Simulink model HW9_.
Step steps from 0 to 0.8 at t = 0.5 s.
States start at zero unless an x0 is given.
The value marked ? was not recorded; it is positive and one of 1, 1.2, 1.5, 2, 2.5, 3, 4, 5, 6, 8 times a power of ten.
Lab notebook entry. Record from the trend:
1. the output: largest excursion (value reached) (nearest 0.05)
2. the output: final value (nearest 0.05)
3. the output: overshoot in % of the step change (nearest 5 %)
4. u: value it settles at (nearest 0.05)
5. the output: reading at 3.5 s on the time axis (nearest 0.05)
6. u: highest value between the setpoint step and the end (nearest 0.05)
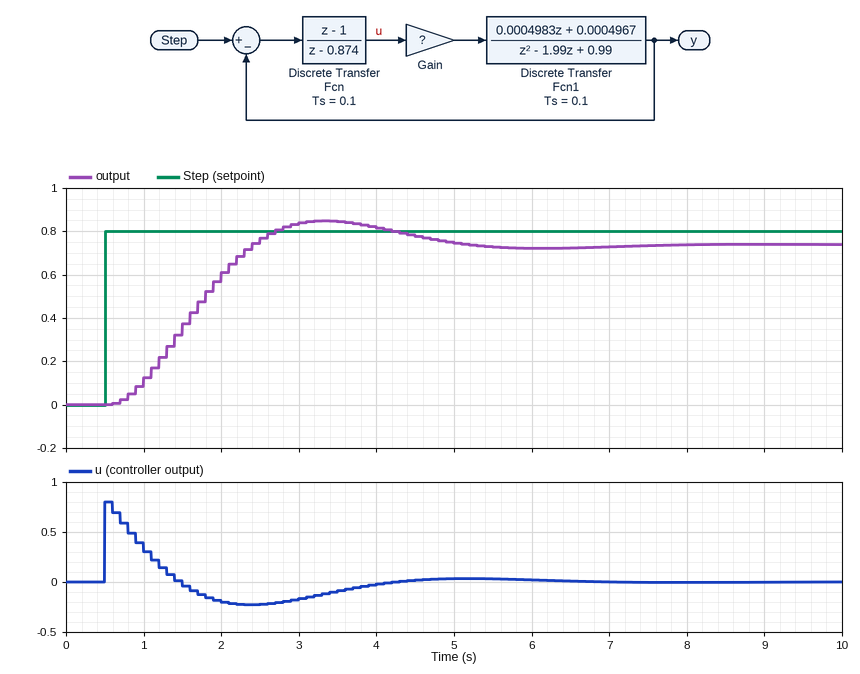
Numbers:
0.85
0.75
15 %
0.00
0.85
0.80
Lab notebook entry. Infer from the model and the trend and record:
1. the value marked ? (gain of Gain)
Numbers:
15
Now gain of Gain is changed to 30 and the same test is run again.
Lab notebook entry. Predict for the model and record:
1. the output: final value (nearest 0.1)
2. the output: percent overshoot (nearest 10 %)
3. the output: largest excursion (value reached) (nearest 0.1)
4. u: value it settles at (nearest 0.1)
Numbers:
0.8
30 %
1.0
0.0
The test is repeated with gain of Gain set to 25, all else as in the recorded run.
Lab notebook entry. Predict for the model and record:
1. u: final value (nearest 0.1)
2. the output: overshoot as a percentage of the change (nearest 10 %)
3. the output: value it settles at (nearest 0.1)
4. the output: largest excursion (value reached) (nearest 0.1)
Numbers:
0.0
30 %
0.8
1.0
